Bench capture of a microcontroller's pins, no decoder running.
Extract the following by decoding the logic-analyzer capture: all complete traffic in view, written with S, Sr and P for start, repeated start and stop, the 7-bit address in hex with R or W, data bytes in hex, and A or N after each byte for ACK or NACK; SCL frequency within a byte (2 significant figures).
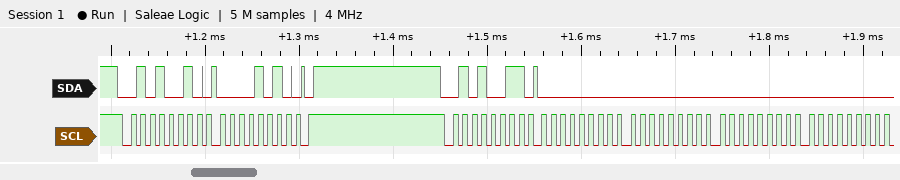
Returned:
S 29W A 0A A P S 29R A 00 A 00 A 00 A 00 A
100 kHz
